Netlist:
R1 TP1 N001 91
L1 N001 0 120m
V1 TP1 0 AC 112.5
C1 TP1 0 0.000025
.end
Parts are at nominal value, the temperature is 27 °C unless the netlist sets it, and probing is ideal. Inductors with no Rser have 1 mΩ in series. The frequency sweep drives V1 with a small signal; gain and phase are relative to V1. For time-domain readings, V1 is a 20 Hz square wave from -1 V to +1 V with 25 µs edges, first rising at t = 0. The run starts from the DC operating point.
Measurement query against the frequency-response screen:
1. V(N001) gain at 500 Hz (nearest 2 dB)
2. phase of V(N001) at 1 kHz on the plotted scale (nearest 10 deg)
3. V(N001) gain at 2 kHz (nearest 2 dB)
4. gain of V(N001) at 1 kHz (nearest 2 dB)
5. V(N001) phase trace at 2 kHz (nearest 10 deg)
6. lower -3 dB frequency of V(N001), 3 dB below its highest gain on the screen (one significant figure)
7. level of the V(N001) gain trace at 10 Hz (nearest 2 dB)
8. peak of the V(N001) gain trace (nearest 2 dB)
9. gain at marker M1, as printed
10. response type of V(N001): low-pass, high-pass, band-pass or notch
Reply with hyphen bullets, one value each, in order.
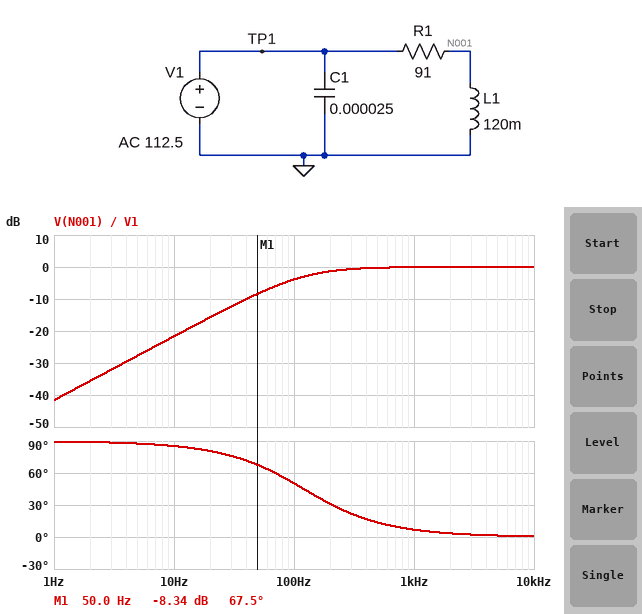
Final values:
- 0 dB
- 10 deg
- 0 dB
- 0 dB
- 0 deg
- 100 Hz
- -22 dB
- 0 dB
- -8.34 dB
- high-pass
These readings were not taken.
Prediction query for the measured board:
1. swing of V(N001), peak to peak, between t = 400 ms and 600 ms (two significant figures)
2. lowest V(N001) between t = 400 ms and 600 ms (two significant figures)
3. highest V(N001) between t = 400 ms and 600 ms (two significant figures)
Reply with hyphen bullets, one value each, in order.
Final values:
- 4.0 V
- -2.0 V
- 2.0 V
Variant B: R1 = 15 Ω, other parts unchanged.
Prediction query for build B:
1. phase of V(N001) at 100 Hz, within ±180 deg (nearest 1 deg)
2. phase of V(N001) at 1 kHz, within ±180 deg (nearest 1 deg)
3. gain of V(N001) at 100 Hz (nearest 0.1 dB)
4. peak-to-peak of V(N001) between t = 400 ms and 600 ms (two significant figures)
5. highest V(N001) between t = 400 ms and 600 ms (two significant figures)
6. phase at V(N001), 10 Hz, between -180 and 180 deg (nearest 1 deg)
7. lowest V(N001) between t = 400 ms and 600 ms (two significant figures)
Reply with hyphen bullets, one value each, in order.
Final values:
- 11 deg
- 1 deg
- -0.2 dB
- 3.8 V
- 1.9 V
- 63 deg
- -1.9 V
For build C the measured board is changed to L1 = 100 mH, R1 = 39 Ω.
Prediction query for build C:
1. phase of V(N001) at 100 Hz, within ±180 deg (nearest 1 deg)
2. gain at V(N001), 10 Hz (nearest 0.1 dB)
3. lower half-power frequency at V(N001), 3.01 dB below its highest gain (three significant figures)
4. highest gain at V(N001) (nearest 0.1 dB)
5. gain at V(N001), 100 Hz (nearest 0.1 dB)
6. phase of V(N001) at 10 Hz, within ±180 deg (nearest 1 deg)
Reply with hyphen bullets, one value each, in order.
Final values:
- 32 deg
- -16.0 dB
- 62.1 Hz
- 0 dB
- -1.4 dB
- 81 deg
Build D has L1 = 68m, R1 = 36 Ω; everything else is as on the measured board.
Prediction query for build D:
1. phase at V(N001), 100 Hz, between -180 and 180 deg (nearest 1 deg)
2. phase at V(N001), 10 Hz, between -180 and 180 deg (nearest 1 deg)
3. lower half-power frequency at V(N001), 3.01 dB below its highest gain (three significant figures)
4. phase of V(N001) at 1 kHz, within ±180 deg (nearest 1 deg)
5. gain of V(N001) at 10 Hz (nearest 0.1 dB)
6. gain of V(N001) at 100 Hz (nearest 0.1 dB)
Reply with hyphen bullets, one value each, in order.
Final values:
- 40 deg
- 83 deg
- 84.3 Hz
- 5 deg
- -18.6 dB
- -2.3 dB
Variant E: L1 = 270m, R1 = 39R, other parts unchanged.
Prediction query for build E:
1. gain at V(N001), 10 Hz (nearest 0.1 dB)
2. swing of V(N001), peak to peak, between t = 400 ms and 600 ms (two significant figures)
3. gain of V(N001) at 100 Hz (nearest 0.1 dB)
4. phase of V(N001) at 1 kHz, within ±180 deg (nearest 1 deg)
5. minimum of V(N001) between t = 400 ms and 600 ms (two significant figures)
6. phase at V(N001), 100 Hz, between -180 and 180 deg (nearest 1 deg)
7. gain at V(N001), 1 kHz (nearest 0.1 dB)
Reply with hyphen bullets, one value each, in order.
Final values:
- -8.0 dB
- 3.9 V
- -0.2 dB
- 1 deg
- -1.9 V
- 13 deg
- 0 dB
